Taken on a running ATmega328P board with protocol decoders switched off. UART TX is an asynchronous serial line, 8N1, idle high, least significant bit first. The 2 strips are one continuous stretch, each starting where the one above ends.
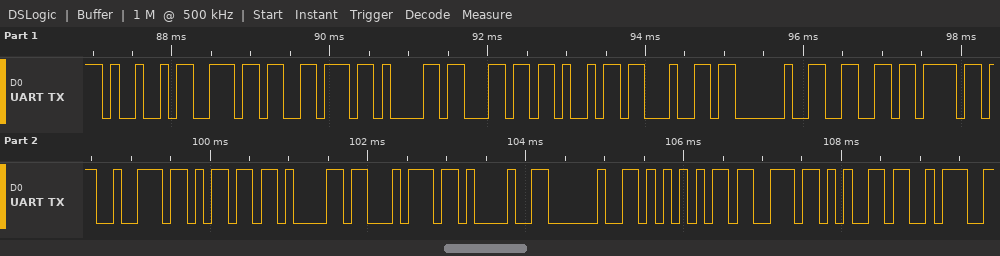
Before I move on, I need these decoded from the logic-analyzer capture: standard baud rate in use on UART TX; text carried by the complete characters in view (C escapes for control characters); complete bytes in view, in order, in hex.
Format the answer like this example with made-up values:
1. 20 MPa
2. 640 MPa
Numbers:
1. 9600 baud
2. "Invalid format! Use:"
3. 49 6E 76 61 6C 69 64 20 66 6F 72 6D 61 74 21 20 55 73 65 3A
